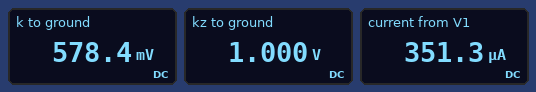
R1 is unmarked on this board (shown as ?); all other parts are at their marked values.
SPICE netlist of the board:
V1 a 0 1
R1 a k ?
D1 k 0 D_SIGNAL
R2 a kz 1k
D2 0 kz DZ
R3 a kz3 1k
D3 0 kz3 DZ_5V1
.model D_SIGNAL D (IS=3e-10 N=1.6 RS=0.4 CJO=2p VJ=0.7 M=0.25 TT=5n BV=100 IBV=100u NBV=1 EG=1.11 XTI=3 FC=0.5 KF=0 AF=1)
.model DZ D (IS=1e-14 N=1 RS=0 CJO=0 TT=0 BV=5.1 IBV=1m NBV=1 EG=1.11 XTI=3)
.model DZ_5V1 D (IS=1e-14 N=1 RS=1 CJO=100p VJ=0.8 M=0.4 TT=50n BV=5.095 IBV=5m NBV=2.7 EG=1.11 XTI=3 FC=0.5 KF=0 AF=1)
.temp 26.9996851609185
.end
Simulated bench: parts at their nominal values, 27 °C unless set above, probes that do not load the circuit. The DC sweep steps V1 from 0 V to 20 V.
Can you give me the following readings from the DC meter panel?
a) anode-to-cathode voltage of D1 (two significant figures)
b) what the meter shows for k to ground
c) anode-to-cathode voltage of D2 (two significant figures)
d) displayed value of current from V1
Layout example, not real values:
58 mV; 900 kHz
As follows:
580 mV; 578.4 mV; -1.0 V; 351.3 µA
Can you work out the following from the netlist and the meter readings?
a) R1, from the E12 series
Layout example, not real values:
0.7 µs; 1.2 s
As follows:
1.2 kΩ
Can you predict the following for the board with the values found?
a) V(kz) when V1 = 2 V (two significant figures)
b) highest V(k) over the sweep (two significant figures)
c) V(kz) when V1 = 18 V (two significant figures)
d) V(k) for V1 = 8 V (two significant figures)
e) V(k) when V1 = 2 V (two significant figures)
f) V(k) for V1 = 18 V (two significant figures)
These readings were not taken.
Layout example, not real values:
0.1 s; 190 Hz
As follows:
2.0 V; 740 mV; 5.2 V; 700 mV; 630 mV; 740 mV
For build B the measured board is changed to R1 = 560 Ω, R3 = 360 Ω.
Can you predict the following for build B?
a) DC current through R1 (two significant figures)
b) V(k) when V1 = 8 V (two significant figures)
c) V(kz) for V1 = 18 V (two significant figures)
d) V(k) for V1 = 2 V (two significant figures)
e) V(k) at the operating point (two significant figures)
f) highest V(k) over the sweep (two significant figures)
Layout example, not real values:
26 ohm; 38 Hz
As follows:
700 µA; 730 mV; 5.2 V; 660 mV; 610 mV; 780 mV
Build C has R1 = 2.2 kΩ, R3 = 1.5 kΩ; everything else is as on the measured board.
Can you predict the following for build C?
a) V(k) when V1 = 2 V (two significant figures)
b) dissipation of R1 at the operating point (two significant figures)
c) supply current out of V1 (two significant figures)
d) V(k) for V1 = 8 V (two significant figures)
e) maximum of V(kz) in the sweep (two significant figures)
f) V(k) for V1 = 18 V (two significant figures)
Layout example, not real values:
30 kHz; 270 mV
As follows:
600 mV; 90 µW; 200 µA; 670 mV; 5.2 V; 710 mV
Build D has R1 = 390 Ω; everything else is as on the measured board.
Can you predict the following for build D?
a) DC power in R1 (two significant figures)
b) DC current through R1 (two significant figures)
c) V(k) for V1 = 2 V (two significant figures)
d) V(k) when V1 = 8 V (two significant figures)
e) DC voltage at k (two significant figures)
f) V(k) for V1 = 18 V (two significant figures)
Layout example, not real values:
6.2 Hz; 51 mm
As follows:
370 µW; 970 µA; 670 mV; 750 mV; 620 mV; 800 mV
